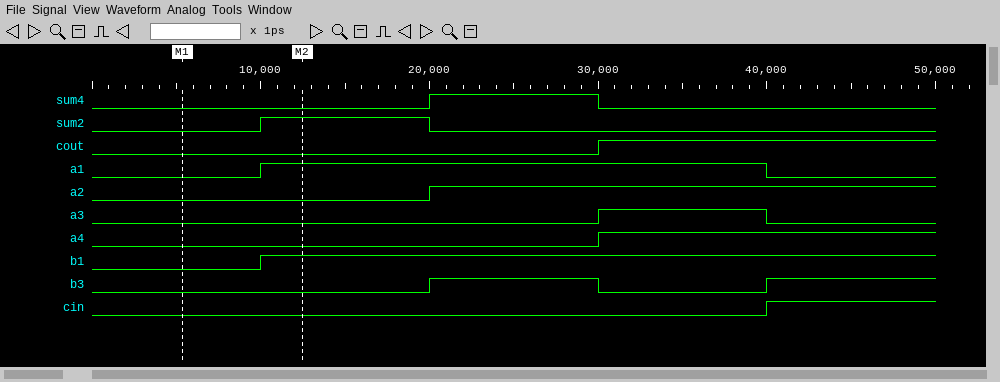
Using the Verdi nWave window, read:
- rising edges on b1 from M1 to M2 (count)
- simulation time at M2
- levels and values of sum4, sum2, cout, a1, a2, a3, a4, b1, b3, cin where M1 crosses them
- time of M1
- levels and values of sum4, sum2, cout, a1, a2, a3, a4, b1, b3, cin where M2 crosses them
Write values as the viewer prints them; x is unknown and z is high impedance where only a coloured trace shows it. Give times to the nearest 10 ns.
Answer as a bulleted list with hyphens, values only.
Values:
- 1
- 10 ns
- sum4=0, sum2=0, cout=0, a1=0, a2=0, a3=0, a4=0, b1=0, b3=0, cin=0
- 10 ns
- sum4=0, sum2=1, cout=0, a1=1, a2=0, a3=0, a4=0, b1=1, b3=0, cin=0
